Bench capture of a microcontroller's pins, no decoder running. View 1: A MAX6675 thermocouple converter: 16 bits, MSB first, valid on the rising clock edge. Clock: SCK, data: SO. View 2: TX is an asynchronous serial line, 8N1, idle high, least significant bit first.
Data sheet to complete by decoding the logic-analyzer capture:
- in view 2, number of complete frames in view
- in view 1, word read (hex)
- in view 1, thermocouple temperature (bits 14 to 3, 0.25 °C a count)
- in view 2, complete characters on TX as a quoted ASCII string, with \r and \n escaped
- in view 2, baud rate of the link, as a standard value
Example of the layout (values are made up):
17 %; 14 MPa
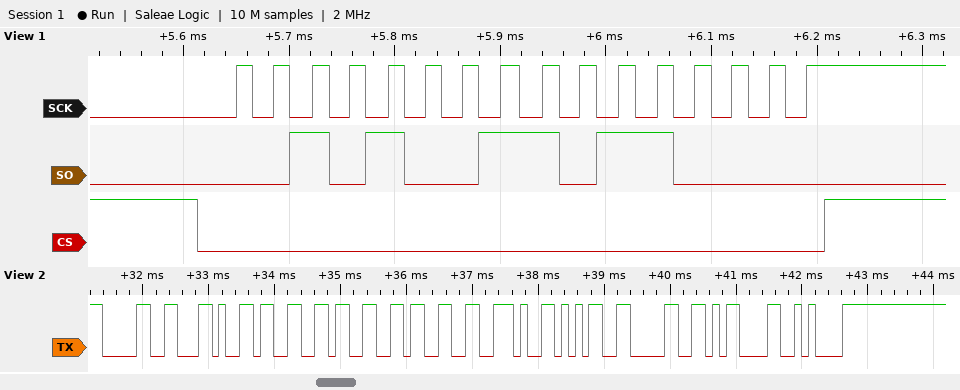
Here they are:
10; 0x29B0; 333.50 °C; "0,333.50\r\n"; 9600 baud
